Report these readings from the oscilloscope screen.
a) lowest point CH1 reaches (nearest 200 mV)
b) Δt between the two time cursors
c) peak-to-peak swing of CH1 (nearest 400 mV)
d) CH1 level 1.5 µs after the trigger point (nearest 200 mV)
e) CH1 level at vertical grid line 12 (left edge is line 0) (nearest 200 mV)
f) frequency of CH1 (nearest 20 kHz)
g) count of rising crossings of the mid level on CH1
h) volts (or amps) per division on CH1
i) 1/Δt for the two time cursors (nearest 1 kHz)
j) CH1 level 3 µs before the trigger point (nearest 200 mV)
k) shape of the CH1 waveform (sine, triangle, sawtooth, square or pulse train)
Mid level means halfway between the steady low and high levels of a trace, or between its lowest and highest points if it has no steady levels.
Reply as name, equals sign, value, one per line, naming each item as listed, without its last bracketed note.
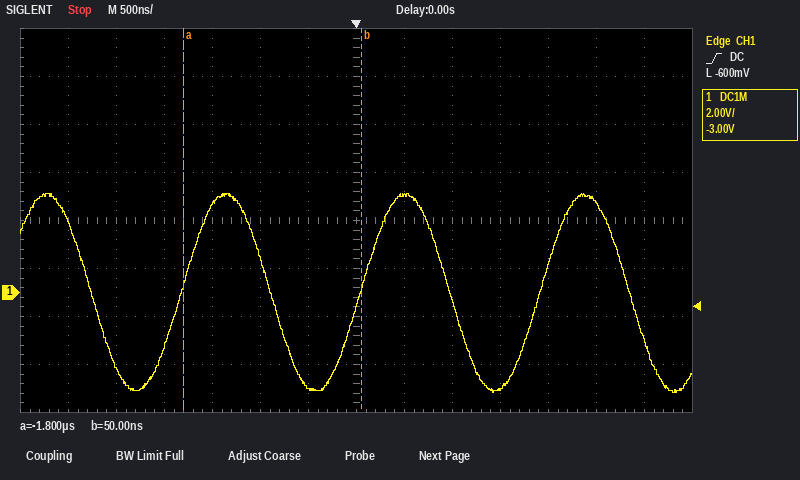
lowest point CH1 reaches = -4.2 V
Δt between the two time cursors = 1.85 µs
peak-to-peak swing of CH1 = 8.4 V
CH1 level 1.5 µs after the trigger point = -4.0 V
CH1 level at vertical grid line 12 (left edge is line 0) = 3.8 V
frequency of CH1 = 540 kHz
count of rising crossings of the mid level on CH1 = 3
volts (or amps) per division on CH1 = 2 V
1/Δt for the two time cursors = 541 kHz
CH1 level 3 µs before the trigger point = 3.0 V
shape of the CH1 waveform = sine
